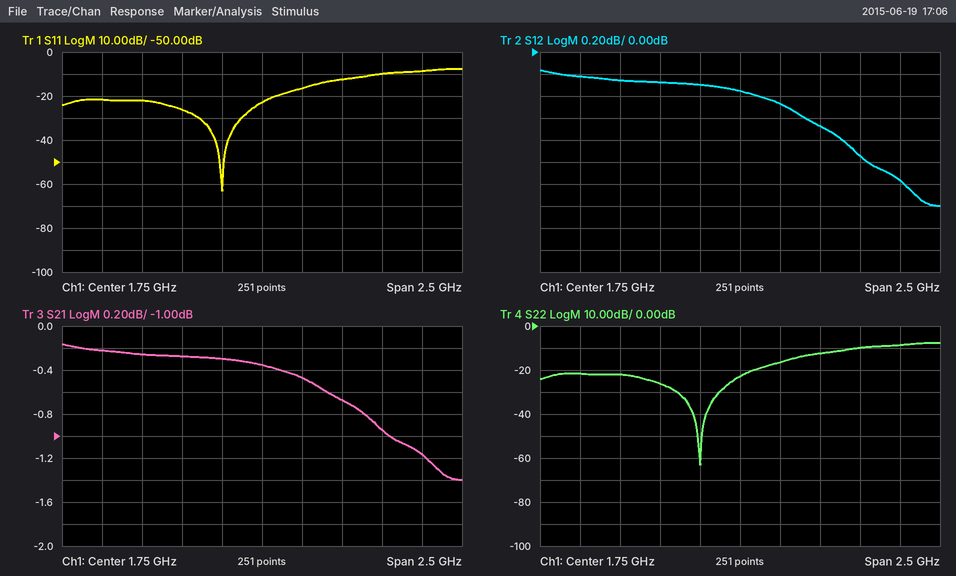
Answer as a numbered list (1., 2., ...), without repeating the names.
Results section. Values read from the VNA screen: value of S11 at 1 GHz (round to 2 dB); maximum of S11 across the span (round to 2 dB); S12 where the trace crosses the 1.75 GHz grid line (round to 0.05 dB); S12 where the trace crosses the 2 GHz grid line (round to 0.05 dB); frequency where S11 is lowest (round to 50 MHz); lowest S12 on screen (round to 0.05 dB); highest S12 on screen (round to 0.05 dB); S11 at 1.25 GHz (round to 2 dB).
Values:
1. -22 dB
2. -8 dB
3. -0.35 dB
4. -0.45 dB
5. 1.50 GHz
6. -1.40 dB
7. -0.15 dB
8. -26 dB
